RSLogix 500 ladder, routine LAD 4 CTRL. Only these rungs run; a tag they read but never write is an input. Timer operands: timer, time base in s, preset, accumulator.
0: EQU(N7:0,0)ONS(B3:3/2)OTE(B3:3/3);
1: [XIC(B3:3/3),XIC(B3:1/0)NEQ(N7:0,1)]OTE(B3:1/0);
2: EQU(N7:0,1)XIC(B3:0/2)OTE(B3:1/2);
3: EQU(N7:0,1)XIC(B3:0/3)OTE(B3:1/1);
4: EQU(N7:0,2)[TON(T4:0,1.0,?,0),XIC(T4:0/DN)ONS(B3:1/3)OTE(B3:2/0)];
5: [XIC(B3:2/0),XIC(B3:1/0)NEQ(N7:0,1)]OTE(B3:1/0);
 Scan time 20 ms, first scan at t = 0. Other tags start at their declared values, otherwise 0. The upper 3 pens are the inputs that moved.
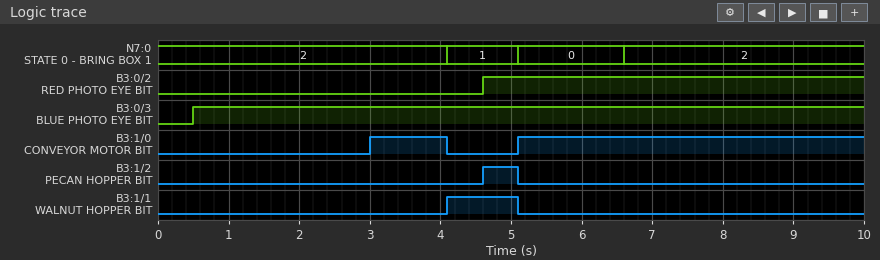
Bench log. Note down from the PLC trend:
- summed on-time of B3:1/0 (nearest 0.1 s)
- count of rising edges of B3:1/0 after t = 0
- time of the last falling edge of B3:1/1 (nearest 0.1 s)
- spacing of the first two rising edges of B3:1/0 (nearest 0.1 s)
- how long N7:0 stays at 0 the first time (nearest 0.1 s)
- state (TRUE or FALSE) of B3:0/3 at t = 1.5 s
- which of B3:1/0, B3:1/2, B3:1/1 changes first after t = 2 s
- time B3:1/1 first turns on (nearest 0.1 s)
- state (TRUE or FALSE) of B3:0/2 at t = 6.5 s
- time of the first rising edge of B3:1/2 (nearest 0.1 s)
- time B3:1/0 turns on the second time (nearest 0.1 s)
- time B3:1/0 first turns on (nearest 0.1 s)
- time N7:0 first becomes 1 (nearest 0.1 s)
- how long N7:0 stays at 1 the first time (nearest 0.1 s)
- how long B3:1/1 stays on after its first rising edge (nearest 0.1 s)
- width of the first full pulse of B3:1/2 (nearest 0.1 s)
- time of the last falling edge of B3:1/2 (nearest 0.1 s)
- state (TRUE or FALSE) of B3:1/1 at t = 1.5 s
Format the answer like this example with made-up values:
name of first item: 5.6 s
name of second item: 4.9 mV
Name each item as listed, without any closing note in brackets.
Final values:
summed on-time of B3:1/0: 6.0 s
count of rising edges of B3:1/0 after t = 0: 2
time of the last falling edge of B3:1/1: 5.1 s
spacing of the first two rising edges of B3:1/0: 2.1 s
how long N7:0 stays at 0 the first time: 1.5 s
state (TRUE or FALSE) of B3:0/3 at t = 1.5 s: TRUE
which of B3:1/0, B3:1/2, B3:1/1 changes first after t = 2 s: B3:1/0
time B3:1/1 first turns on: 4.1 s
state (TRUE or FALSE) of B3:0/2 at t = 6.5 s: TRUE
time of the first rising edge of B3:1/2: 4.6 s
time B3:1/0 turns on the second time: 5.1 s
time B3:1/0 first turns on: 3.0 s
time N7:0 first becomes 1: 4.1 s
how long N7:0 stays at 1 the first time: 1.0 s
how long B3:1/1 stays on after its first rising edge: 1.0 s
width of the first full pulse of B3:1/2: 0.5 s
time of the last falling edge of B3:1/2: 5.1 s
state (TRUE or FALSE) of B3:1/1 at t = 1.5 s: FALSE
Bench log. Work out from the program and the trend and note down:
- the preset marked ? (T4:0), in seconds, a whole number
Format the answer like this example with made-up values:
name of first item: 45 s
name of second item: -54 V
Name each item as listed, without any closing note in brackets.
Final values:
the preset marked ? (T4:0), in seconds, a whole number: 3 s
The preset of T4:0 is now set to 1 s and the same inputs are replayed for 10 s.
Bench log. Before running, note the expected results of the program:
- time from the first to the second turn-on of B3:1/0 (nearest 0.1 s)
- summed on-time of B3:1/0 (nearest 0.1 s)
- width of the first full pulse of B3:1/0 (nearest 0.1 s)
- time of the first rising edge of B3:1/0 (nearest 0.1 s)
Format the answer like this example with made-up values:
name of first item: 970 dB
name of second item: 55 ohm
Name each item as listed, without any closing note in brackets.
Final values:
time from the first to the second turn-on of B3:1/0: 4.1 s
summed on-time of B3:1/0: 8.0 s
width of the first full pulse of B3:1/0: 3.1 s
time of the first rising edge of B3:1/0: 1.0 s
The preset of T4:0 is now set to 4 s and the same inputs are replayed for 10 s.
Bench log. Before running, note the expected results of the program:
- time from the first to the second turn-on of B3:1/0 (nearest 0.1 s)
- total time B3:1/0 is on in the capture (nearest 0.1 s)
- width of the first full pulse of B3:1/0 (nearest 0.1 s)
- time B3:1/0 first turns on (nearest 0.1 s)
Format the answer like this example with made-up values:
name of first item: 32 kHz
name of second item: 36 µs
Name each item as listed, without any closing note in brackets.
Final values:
time from the first to the second turn-on of B3:1/0: 1.1 s
total time B3:1/0 is on in the capture: 5.0 s
width of the first full pulse of B3:1/0: 0.1 s
time B3:1/0 first turns on: 4.0 s
